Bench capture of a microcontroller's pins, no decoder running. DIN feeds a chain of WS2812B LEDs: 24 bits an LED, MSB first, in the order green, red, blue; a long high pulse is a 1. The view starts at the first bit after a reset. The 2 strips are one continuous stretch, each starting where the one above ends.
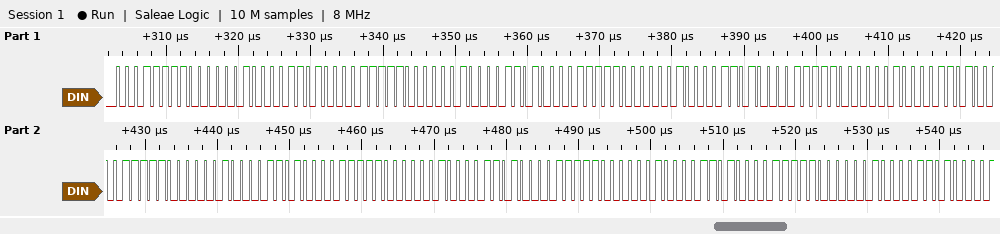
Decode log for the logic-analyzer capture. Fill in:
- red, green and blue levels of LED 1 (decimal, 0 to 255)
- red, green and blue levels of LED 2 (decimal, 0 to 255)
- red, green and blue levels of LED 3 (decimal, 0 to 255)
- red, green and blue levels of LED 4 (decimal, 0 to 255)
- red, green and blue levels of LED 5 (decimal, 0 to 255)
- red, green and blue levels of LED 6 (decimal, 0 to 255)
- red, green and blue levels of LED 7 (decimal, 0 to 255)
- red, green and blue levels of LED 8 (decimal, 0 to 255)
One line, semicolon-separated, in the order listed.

2, 31, 26; 2, 31, 26; 2, 31, 26; 2, 31, 26; 2, 31, 26; 2, 31, 26; 2, 31, 26; 2, 31, 26
